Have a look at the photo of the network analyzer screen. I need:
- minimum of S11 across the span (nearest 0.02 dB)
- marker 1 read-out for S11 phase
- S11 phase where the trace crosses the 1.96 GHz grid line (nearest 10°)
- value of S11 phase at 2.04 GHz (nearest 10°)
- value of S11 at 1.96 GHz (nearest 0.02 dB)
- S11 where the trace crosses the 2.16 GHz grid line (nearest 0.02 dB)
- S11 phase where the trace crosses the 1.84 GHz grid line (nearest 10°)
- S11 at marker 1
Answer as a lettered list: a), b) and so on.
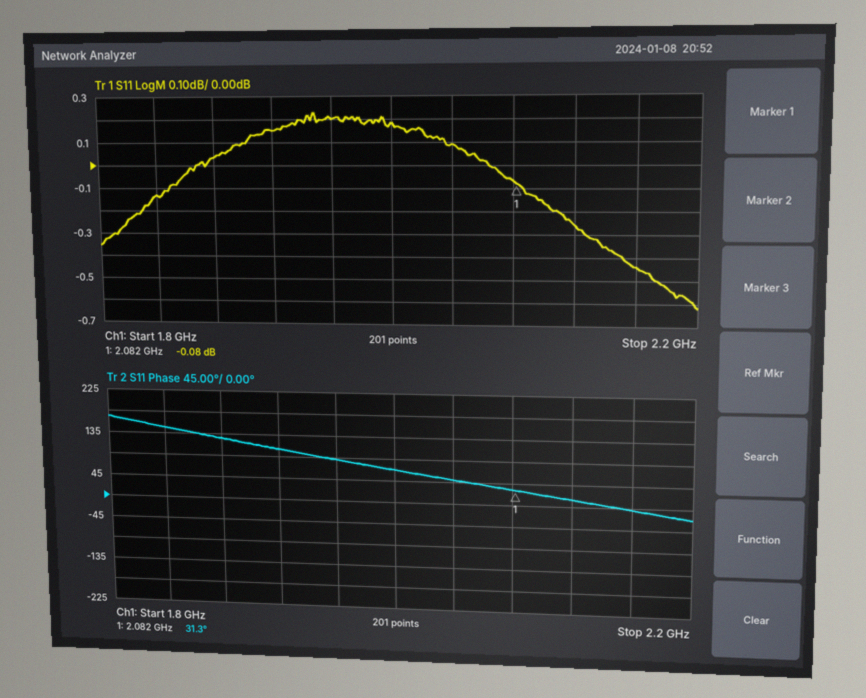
a) -0.62 dB
b) 31.3°
c) 90°
d) 50°
e) 0.20 dB
f) -0.44 dB
g) 150°
h) -0.08 dB
